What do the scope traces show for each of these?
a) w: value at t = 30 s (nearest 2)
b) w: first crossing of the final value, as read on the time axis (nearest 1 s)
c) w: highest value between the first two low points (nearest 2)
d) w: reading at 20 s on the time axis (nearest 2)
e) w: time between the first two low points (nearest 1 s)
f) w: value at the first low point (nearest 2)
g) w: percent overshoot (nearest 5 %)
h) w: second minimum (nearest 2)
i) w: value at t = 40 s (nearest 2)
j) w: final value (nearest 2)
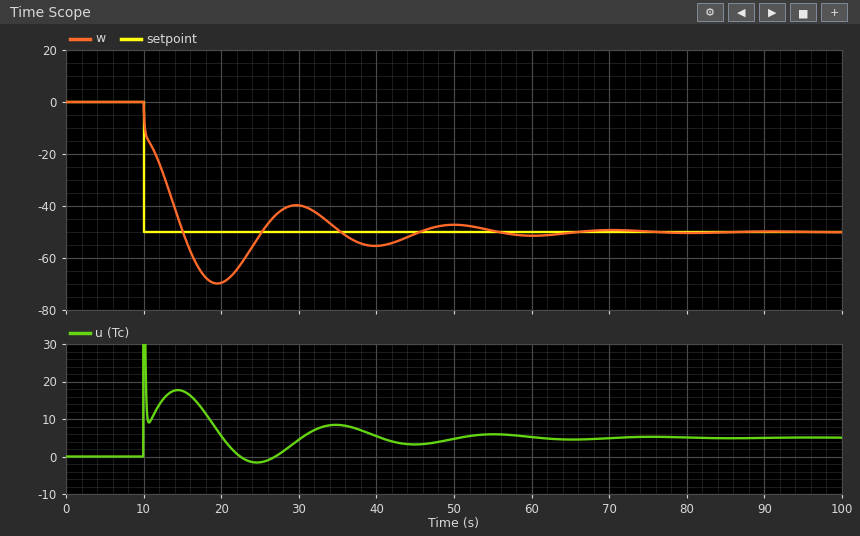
-40
15 s
-40
-70
20 s
-70
40 %
-56
-56
-50
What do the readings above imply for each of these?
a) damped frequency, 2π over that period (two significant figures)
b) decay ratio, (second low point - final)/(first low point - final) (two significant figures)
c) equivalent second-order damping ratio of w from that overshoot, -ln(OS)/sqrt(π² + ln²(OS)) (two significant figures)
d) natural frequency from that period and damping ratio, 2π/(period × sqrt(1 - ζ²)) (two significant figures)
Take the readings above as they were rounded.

0.31 rad/s
0.30
0.28
0.33 rad/s
